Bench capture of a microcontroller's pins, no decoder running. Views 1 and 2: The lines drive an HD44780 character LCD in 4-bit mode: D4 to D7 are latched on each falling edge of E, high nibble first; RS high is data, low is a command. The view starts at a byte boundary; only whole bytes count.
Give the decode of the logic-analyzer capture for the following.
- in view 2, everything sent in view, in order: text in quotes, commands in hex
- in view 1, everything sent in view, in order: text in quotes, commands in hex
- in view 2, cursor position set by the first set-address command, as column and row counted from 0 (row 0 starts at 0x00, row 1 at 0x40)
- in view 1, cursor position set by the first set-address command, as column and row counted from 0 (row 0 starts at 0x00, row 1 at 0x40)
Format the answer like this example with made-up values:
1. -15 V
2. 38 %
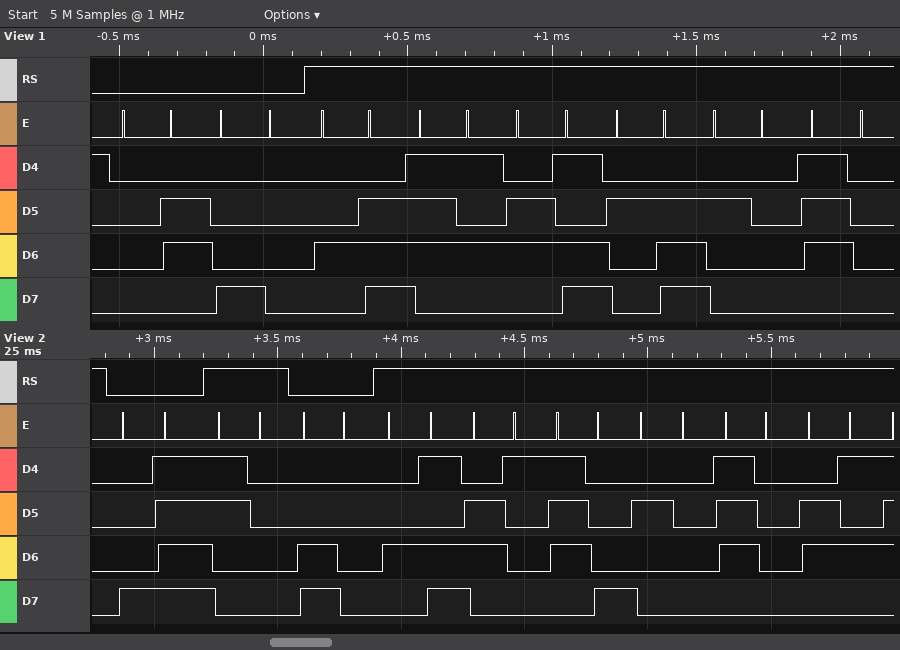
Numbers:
1. 0x8F "0" 0xC0 "Max pe"
2. 0x06 0x80 "Num. p"
3. column 15, row 0
4. column 0, row 0
